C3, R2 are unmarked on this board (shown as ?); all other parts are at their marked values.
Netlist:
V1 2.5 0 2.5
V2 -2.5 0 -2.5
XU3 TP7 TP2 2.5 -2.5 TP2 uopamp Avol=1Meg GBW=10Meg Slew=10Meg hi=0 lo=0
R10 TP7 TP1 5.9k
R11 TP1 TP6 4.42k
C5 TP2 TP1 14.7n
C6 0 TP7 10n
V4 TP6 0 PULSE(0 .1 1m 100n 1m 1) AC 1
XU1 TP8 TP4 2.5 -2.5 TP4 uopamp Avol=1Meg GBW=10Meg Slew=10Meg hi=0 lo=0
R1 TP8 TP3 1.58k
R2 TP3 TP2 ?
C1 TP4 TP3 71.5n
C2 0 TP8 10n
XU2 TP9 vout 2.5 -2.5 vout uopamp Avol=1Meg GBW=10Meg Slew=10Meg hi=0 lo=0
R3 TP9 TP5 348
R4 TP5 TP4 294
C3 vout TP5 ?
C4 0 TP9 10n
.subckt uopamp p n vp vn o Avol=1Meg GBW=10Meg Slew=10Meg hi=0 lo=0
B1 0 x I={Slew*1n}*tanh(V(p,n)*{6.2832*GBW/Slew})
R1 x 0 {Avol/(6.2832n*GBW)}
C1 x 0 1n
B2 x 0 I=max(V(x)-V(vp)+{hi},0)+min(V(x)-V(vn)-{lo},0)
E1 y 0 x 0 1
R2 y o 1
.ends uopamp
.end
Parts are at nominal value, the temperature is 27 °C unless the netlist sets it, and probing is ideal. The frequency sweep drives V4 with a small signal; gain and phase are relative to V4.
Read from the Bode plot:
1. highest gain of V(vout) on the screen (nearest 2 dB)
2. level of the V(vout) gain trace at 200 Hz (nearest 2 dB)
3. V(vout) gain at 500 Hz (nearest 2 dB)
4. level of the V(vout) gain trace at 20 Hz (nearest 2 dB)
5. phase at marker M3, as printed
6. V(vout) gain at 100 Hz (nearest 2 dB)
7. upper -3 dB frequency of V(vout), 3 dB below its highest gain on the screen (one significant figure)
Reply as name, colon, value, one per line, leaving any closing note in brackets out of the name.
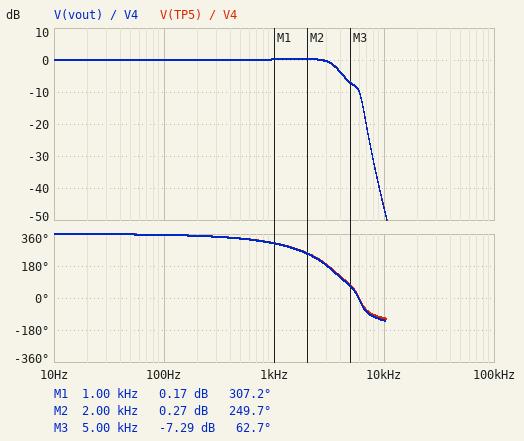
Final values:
highest gain of V(vout) on the screen: 0 dB
level of the V(vout) gain trace at 200 Hz: 0 dB
V(vout) gain at 500 Hz: 0 dB
level of the V(vout) gain trace at 20 Hz: 0 dB
phase at marker M3, as printed: 62.7 deg
V(vout) gain at 100 Hz: 0 dB
upper -3 dB frequency of V(vout), 3 dB below its highest gain on the screen: 4 kHz
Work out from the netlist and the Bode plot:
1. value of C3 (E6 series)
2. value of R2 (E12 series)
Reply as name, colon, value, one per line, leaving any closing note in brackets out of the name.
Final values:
value of C3: 680 nF
value of R2: 1.8 kΩ
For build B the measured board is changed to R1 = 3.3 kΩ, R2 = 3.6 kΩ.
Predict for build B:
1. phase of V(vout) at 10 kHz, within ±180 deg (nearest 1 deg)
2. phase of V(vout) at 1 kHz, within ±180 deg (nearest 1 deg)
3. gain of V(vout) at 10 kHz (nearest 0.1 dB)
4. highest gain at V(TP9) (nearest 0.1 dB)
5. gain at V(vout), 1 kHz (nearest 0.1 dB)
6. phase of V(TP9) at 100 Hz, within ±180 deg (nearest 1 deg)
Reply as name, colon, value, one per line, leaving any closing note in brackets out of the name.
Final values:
phase of V(vout) at 10 kHz, within ±180 deg: -135 deg
phase of V(vout) at 1 kHz, within ±180 deg: -73 deg
gain of V(vout) at 10 kHz: -59.3 dB
highest gain at V(TP9): 2.4 dB
gain at V(vout), 1 kHz: 1.7 dB
phase of V(TP9) at 100 Hz, within ±180 deg: -6 deg
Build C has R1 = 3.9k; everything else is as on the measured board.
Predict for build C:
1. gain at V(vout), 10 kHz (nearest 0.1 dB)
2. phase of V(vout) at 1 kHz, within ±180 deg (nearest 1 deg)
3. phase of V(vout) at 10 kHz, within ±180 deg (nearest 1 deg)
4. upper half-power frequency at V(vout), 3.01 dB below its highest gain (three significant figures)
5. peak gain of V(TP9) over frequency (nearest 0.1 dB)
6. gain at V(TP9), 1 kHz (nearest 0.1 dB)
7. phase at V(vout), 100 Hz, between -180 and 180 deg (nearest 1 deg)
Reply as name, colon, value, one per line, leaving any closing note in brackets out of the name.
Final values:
gain at V(vout), 10 kHz: -54.6 dB
phase of V(vout) at 1 kHz, within ±180 deg: -64 deg
phase of V(vout) at 10 kHz, within ±180 deg: -132 deg
upper half-power frequency at V(vout), 3.01 dB below its highest gain: 2.45 kHz
peak gain of V(TP9) over frequency: 1.4 dB
gain at V(TP9), 1 kHz: 0.8 dB
phase at V(vout), 100 Hz, between -180 and 180 deg: -6 deg
